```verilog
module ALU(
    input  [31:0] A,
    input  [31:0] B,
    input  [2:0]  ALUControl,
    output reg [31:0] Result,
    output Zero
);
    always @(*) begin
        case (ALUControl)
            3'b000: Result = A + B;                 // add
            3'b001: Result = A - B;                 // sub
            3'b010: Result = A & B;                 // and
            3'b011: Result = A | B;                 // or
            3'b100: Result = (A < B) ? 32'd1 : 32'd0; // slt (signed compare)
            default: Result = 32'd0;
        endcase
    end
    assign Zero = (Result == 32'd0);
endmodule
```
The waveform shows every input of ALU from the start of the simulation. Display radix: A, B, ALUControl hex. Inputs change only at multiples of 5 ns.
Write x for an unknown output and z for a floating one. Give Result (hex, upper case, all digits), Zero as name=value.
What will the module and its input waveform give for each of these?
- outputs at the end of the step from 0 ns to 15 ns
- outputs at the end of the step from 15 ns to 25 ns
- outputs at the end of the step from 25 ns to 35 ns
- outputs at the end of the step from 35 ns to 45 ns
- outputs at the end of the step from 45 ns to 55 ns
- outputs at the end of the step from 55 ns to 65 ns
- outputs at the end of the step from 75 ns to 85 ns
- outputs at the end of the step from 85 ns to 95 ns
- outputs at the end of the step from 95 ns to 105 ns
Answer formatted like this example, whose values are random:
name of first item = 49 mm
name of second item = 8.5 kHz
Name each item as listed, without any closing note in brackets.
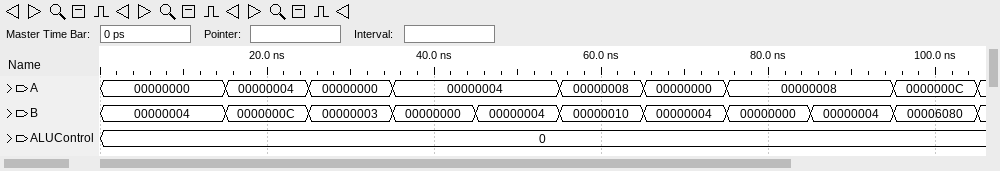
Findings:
outputs at the end of the step from 0 ns to 15 ns = Result=00000004, Zero=0
outputs at the end of the step from 15 ns to 25 ns = Result=00000010, Zero=0
outputs at the end of the step from 25 ns to 35 ns = Result=00000003, Zero=0
outputs at the end of the step from 35 ns to 45 ns = Result=00000004, Zero=0
outputs at the end of the step from 45 ns to 55 ns = Result=00000008, Zero=0
outputs at the end of the step from 55 ns to 65 ns = Result=00000018, Zero=0
outputs at the end of the step from 75 ns to 85 ns = Result=00000008, Zero=0
outputs at the end of the step from 85 ns to 95 ns = Result=0000000C, Zero=0
outputs at the end of the step from 95 ns to 105 ns = Result=0000608C, Zero=0
